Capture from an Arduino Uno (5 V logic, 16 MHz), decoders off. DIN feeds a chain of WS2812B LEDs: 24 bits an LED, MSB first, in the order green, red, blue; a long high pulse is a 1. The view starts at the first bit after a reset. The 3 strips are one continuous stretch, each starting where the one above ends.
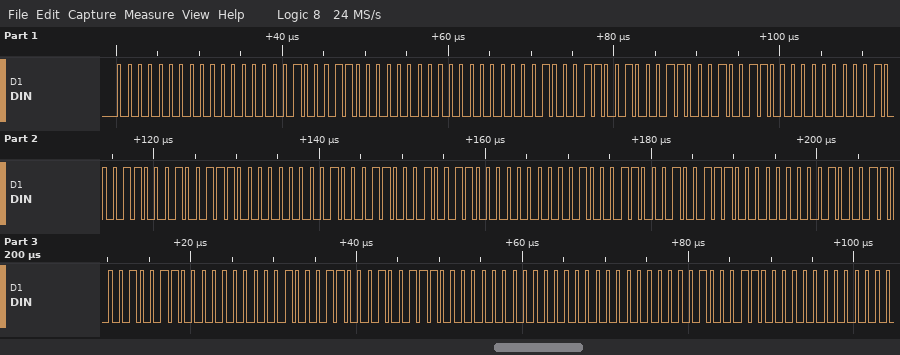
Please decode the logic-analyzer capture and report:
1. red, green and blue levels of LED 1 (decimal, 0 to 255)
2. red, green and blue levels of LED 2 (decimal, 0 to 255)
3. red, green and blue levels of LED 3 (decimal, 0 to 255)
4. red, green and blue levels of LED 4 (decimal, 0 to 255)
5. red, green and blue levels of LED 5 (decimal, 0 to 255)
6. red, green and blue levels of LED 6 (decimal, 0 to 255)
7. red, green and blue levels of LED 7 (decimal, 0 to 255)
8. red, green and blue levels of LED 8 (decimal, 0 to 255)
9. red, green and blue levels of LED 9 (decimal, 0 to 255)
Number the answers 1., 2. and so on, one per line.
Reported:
1. 0, 0, 70
2. 0, 0, 70
3. 38, 70, 0
4. 39, 70, 0
5. 38, 70, 0
6. 39, 70, 0
7. 38, 70, 0
8. 39, 70, 0
9. 0, 0, 70
